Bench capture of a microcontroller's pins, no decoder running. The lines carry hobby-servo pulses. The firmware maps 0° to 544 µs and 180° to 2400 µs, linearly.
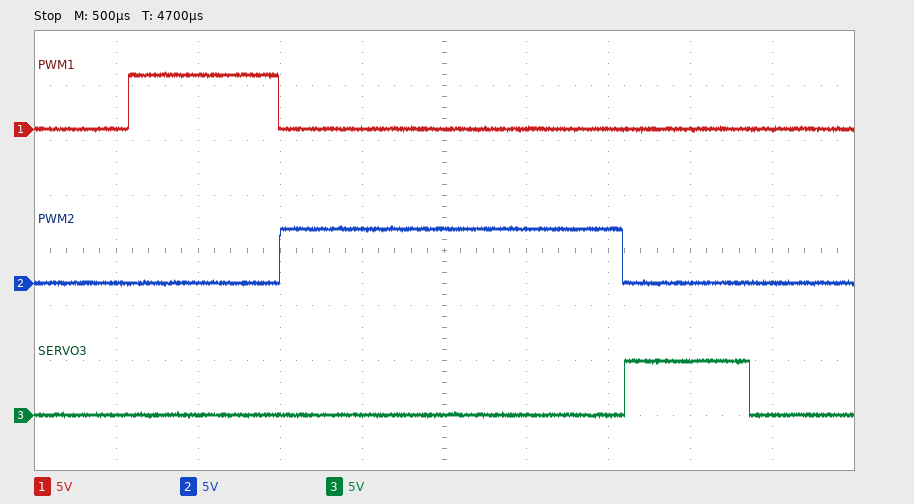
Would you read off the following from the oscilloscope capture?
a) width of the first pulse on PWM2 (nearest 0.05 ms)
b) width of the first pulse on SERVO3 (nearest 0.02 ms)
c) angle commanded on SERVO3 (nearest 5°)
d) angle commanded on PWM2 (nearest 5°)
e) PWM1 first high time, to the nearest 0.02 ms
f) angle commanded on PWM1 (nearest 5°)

2.10 ms
0.76 ms
20°
150°
0.92 ms
35°
